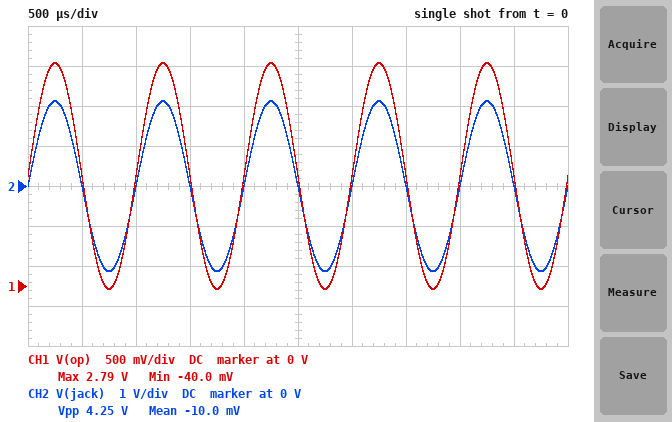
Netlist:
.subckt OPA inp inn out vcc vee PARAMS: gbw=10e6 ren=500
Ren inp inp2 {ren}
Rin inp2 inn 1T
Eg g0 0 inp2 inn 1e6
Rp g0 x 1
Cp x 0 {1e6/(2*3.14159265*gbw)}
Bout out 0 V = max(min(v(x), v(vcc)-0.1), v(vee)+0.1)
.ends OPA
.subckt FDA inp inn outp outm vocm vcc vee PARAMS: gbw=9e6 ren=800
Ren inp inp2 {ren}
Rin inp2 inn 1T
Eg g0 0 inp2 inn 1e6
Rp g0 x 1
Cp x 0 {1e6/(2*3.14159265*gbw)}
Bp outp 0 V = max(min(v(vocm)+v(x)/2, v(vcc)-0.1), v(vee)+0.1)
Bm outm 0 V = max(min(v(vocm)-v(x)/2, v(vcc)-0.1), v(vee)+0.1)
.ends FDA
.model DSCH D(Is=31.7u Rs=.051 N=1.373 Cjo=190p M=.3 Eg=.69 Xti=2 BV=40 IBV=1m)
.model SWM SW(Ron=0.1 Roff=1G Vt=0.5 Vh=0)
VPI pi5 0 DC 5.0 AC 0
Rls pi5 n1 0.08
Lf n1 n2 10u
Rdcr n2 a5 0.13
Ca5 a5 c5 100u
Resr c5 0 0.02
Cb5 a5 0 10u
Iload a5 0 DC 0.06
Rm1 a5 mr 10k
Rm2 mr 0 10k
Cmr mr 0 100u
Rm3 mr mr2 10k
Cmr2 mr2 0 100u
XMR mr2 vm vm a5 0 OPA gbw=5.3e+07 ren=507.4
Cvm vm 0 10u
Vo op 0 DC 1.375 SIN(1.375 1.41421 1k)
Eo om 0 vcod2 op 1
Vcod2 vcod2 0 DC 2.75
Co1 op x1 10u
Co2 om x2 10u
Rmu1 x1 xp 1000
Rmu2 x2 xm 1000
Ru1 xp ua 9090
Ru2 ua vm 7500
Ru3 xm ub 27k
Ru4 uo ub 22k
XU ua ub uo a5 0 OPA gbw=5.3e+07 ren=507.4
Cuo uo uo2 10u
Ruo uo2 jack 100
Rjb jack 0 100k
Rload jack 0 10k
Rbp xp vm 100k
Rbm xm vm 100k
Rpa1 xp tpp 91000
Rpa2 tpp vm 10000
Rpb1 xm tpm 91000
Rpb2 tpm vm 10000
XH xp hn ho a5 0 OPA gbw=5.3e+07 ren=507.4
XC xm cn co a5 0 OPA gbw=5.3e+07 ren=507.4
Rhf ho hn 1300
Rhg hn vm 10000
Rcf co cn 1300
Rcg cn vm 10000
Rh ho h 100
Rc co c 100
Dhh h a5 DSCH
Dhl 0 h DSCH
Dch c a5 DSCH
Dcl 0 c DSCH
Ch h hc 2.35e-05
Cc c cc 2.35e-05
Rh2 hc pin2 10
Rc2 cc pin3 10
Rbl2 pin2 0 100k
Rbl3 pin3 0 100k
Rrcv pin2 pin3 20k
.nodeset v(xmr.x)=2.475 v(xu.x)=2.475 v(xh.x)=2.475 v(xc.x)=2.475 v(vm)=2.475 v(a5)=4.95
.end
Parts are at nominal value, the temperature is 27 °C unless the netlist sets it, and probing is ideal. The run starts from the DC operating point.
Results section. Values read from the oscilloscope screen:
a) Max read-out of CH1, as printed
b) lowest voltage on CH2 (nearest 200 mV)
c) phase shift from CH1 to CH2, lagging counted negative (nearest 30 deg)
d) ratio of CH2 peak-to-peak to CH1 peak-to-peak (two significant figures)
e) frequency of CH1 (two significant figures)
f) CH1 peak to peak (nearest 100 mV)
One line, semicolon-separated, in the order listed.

2.79 V; -2.2 V; 0 deg; 1.5; 1.0 kHz; 2.8 V
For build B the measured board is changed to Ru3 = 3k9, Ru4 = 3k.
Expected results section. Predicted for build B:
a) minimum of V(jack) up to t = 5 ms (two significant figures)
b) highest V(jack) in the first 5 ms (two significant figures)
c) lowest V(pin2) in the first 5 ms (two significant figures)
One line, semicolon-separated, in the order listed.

-1.8 V; 1.8 V; -1.5 V
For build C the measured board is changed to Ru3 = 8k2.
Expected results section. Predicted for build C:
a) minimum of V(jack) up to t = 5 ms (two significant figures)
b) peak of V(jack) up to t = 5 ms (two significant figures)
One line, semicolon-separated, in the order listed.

-2.4 V; 2.4 V
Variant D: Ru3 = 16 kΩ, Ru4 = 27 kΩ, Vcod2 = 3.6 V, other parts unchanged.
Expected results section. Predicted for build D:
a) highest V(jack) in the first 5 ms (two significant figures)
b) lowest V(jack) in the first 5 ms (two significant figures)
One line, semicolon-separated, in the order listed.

2.4 V; -2.4 V
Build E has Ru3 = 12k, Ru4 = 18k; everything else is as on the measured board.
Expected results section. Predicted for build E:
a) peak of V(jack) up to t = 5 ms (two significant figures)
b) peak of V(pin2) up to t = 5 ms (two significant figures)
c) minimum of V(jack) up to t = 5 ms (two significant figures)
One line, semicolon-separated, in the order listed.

2.4 V; 1.5 V; -2.4 V
